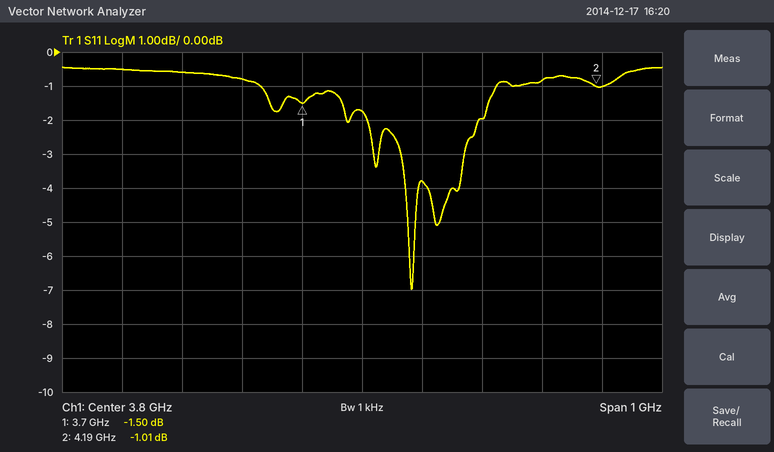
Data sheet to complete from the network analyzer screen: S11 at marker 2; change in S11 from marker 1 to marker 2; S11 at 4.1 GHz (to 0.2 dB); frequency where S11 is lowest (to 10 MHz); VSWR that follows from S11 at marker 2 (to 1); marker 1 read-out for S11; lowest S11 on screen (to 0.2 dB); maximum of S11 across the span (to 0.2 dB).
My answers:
-1.01 dB
0.49 dB
-0.8 dB
3.88 GHz
17
-1.50 dB
-7.0 dB
-0.4 dB
